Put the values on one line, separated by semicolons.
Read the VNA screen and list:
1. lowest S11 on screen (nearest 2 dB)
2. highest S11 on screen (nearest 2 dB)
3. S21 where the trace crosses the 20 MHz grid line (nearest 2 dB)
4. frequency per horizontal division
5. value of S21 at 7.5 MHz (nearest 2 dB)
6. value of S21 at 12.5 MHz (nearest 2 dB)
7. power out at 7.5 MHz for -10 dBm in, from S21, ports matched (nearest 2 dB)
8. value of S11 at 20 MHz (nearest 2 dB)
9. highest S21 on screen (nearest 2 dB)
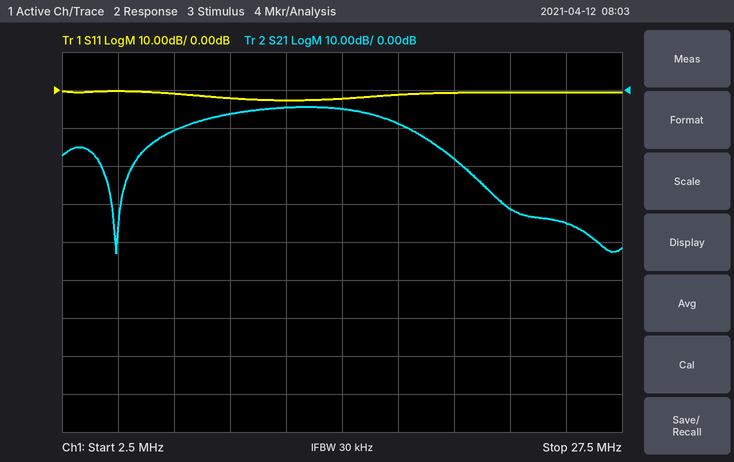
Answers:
-2 dB; 0 dB; -18 dB; 2.5 MHz; -10 dB; -4 dB; -20 dBm; 0 dB; -4 dB
